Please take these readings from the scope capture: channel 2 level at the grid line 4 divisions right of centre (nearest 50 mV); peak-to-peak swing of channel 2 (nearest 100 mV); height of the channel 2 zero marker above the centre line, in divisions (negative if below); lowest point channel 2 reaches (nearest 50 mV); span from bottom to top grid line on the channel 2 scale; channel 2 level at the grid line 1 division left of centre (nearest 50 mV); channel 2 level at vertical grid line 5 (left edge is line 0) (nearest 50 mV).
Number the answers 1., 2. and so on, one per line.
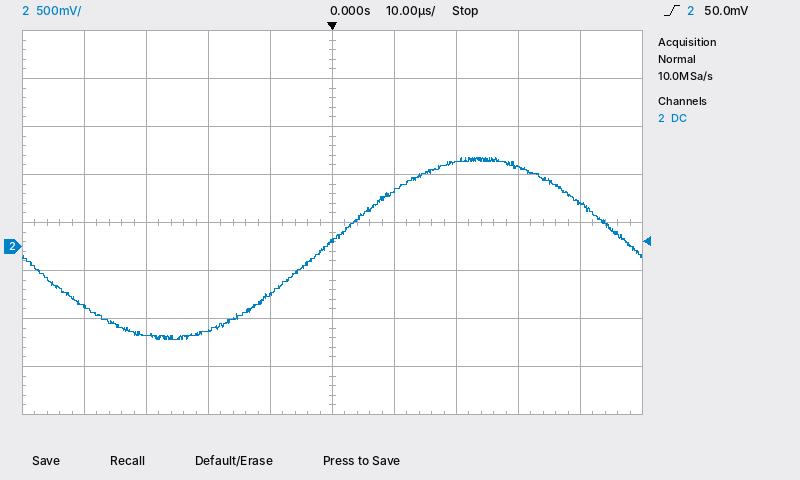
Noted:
1. 450 mV
2. 1.90 V
3. -0.5 div
4. -950 mV
5. 4 V
6. -500 mV
7. 50 mV
